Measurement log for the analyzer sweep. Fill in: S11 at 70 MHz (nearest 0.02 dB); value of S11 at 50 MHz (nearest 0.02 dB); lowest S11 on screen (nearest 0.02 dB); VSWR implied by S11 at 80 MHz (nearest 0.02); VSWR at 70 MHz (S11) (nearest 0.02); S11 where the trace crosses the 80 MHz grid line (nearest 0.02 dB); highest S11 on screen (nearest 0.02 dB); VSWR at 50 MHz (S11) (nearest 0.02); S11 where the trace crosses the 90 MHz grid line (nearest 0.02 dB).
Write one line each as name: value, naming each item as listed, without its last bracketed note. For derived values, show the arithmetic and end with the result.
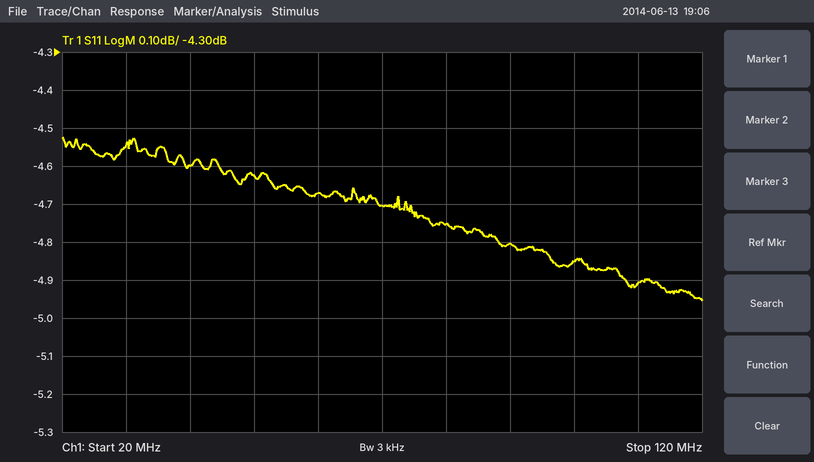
S11 at 70 MHz: -4.70 dB
value of S11 at 50 MHz: -4.62 dB
lowest S11 on screen: -4.96 dB
VSWR implied by S11 at 80 MHz: |Γ| = 10^(-4.76/20) = 0.5781; VSWR = (1 + 0.5781)/(1 − 0.5781) ≈ 3.74
VSWR at 70 MHz (S11): |Γ| = 10^(-4.7/20) = 0.5821; VSWR = (1 + 0.5821)/(1 − 0.5821) ≈ 3.79, so 3.78 to the nearest 0.02
S11 where the trace crosses the 80 MHz grid line: -4.76 dB
highest S11 on screen: -4.52 dB
VSWR at 50 MHz (S11): |Γ| = 10^(-4.62/20) = 0.5875; VSWR = (1 + 0.5875)/(1 − 0.5875) ≈ 3.85, so 3.84 to the nearest 0.02
S11 where the trace crosses the 90 MHz grid line: -4.80 dB
